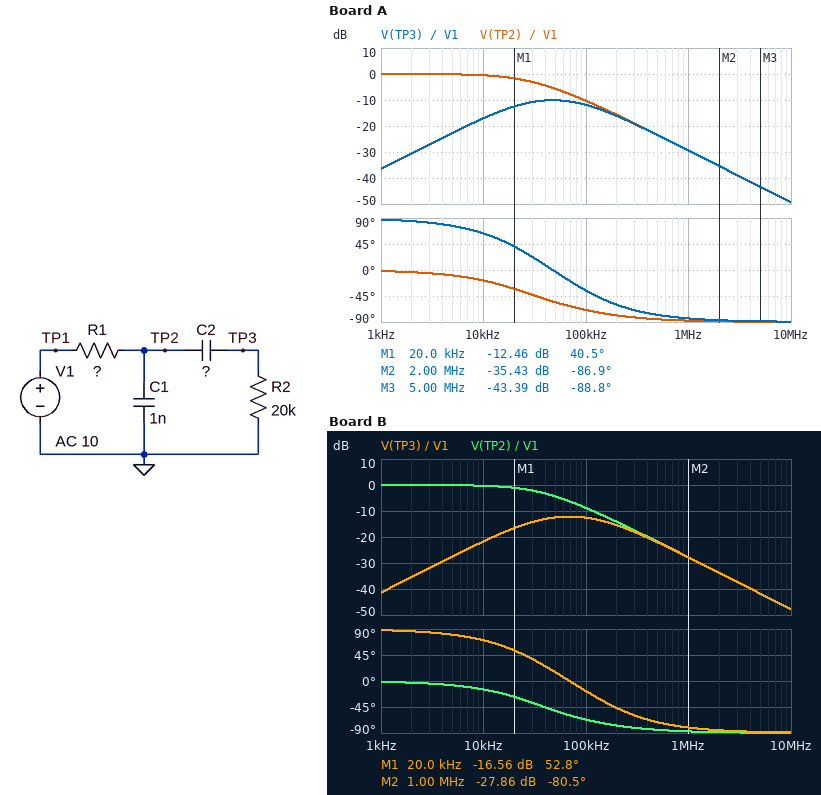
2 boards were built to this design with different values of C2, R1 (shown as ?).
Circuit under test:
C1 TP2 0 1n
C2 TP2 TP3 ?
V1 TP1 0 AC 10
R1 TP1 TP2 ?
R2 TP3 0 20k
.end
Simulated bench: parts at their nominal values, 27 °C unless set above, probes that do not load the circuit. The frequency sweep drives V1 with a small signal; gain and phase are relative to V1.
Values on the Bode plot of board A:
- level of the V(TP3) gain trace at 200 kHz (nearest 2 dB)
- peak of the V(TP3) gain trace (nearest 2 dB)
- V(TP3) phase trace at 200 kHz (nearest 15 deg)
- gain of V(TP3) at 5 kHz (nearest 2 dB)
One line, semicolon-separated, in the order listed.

-16 dB; -10 dB; -60 deg; -22 dB
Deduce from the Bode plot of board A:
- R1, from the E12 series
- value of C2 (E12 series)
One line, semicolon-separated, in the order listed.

4.7 kΩ; 120 pF
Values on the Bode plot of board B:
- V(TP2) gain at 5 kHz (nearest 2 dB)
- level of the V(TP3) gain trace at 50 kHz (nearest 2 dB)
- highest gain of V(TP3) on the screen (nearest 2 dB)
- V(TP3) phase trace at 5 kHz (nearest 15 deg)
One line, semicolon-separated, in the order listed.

0 dB; -12 dB; -12 dB; 75 deg
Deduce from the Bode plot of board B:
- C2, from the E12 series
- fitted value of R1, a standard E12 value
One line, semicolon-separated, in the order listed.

68 pF; 3.9 kΩ
